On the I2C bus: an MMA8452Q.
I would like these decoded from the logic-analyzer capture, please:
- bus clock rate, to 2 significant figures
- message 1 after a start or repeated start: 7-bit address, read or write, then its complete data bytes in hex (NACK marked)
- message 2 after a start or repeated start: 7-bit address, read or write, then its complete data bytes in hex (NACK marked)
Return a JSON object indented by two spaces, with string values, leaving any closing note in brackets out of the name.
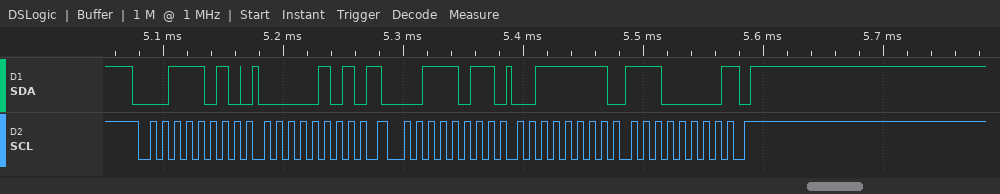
{
  "bus clock rate, to 2 significant figures": "100 kHz",
  "message 1 after a start or repeated start: 7-bit address, read or write, then its complete data bytes in hex": "0x1D write: 05",
  "message 2 after a start or repeated start: 7-bit address, read or write, then its complete data bytes in hex": "0x1D read: 3F E0 NACK"
}
